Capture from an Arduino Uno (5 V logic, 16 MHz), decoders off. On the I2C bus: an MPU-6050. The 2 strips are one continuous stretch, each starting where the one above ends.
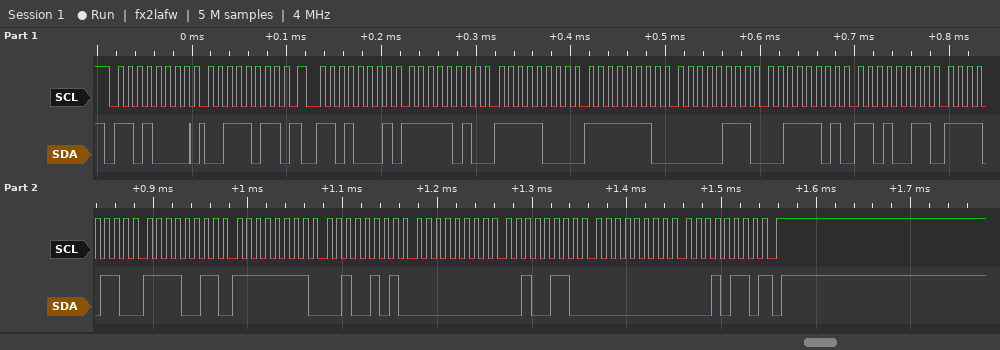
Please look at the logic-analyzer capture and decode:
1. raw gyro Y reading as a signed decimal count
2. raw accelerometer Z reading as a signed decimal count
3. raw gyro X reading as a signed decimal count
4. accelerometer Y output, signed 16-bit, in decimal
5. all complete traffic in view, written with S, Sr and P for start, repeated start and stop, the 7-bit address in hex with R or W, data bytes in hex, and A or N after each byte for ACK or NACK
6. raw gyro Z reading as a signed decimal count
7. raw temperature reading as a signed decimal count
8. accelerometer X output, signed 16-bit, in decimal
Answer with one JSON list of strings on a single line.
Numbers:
["38", "15827", "-219", "-505", "S 68W A 3B A Sr 68R A FA A F8 A FE A 07 A 3D A D3 A F6 A F3 A FF A 25 A 00 A 26 A 00 A 16 N P", "22", "-2317", "-1288"]
